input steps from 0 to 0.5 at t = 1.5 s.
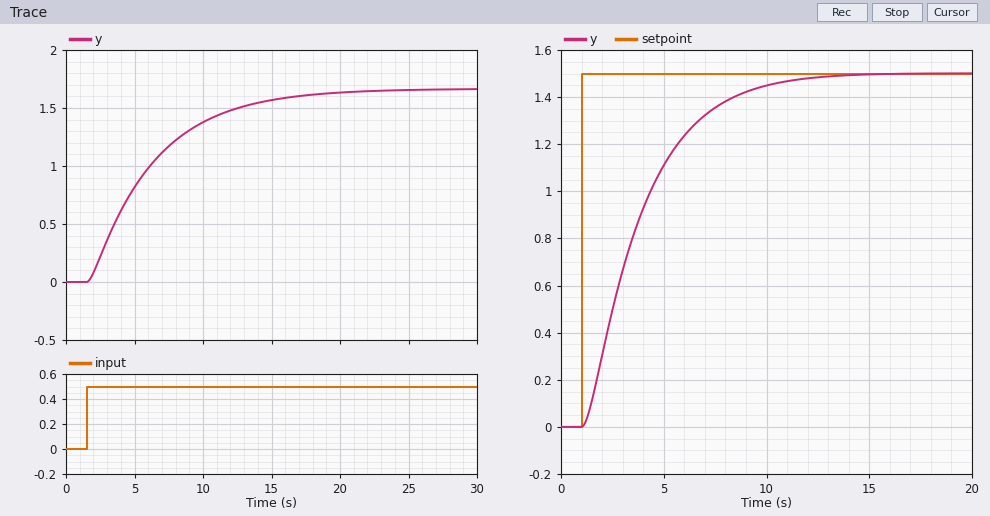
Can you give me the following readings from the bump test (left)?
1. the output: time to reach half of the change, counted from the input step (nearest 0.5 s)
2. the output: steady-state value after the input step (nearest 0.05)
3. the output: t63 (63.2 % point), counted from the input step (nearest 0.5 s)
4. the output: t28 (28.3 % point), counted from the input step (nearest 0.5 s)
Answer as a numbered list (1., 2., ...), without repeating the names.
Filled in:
1. 3.5 s
2. 1.65
3. 5.0 s
4. 2.0 s
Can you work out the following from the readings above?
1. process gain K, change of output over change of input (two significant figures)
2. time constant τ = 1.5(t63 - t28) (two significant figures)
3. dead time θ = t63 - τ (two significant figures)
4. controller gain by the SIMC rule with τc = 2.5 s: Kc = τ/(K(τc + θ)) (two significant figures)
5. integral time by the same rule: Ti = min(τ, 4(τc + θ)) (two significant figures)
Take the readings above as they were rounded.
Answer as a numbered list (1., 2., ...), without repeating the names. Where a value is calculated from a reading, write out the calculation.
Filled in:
1. (1.65 - 0) / 0.5 = 3.3
2. 1.5 × (5 - 2) = 4.5 s
3. 5 - 4.5 = 0.50 s
4. 4.5 / (3.3 × (2.5 + 0.5)) = 0.45
5. min(4.5, 4 × (2.5 + 0.5)) = 4.5 s
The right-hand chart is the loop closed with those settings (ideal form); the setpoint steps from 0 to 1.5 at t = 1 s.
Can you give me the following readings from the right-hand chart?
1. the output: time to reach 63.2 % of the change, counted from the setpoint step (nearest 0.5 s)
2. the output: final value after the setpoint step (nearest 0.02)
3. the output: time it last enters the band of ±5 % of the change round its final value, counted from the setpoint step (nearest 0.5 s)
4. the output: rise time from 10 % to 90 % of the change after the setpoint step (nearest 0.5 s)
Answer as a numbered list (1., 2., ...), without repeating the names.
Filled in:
1. 3.0 s
2. 1.50
3. 8.0 s
4. 6.0 s
